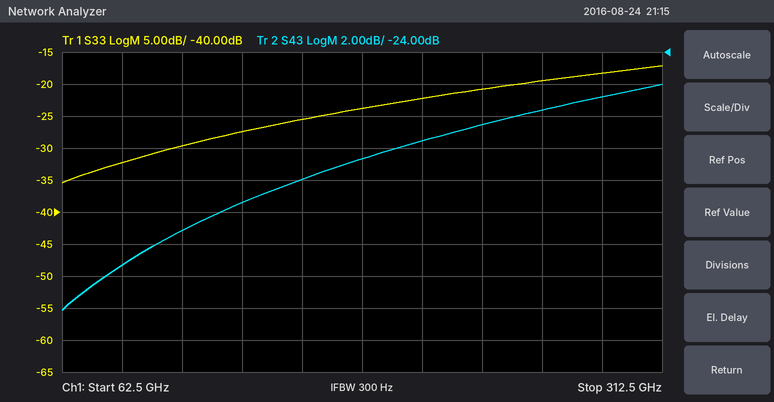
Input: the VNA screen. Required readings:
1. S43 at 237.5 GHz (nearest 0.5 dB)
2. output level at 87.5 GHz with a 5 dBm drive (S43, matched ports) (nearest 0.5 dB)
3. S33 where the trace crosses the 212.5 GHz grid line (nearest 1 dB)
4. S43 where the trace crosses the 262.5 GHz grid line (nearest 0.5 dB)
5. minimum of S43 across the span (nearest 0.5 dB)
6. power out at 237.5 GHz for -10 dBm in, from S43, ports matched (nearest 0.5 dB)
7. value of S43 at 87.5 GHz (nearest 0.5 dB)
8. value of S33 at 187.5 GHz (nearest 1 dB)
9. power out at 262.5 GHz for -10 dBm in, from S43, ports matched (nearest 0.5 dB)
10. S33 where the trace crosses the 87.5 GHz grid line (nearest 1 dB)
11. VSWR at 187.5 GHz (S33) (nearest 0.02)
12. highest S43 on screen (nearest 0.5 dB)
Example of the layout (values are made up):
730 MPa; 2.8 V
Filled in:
-28.5 dB; -32.5 dBm; -22 dB; -27.5 dB; -40.0 dB; -38.5 dBm; -37.5 dB; -24 dB; -37.5 dBm; -32 dB; 1.14; -26.0 dB
